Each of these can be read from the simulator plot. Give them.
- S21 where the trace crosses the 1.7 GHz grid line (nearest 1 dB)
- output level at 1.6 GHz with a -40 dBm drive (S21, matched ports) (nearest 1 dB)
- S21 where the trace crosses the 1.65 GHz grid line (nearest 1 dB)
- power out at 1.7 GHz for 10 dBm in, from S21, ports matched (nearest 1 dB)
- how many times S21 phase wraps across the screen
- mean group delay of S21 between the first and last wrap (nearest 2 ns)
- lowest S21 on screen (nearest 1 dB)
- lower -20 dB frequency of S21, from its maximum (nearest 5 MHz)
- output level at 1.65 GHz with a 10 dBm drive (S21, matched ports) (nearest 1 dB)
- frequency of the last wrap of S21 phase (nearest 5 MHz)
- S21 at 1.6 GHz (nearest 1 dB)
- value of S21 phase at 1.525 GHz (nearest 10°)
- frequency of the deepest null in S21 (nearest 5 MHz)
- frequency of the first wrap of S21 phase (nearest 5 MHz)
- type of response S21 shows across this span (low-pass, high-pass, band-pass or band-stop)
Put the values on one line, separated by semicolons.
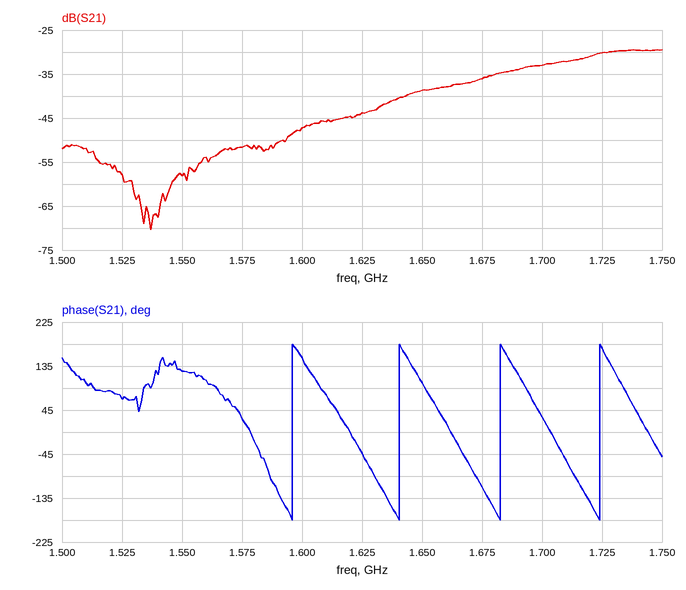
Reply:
-33 dB; -87 dBm; -39 dB; -23 dBm; 4; 24 ns; -70 dB; 1.595 GHz; -29 dBm; 1.725 GHz; -47 dB; 70°; 1.535 GHz; 1.595 GHz; high-pass
